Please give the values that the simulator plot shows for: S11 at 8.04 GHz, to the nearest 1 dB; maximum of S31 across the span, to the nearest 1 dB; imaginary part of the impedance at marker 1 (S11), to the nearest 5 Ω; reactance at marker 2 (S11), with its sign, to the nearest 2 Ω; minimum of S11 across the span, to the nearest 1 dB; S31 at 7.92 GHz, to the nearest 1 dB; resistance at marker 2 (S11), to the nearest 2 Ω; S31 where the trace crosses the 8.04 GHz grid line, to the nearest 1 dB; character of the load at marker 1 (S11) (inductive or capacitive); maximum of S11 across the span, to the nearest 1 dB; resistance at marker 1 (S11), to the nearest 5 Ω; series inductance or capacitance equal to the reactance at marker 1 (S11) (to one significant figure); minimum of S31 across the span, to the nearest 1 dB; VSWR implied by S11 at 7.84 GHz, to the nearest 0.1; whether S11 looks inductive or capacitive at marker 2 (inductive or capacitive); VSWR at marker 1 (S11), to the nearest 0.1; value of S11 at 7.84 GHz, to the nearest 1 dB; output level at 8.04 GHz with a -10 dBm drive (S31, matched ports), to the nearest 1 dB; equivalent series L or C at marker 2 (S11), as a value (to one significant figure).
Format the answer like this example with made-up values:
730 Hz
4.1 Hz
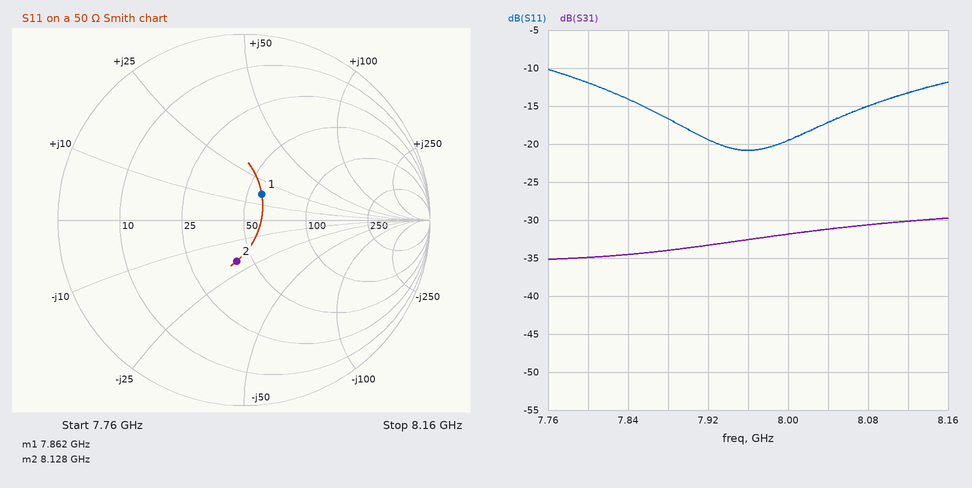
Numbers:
-17 dB
-30 dB
+15 Ω
-20 Ω
-21 dB
-33 dB
42 Ω
-31 dB
inductive
-10 dB
60 Ω
300 pH
-35 dB
1.5
capacitive
1.4
-14 dB
-41 dBm
1.0 pF
